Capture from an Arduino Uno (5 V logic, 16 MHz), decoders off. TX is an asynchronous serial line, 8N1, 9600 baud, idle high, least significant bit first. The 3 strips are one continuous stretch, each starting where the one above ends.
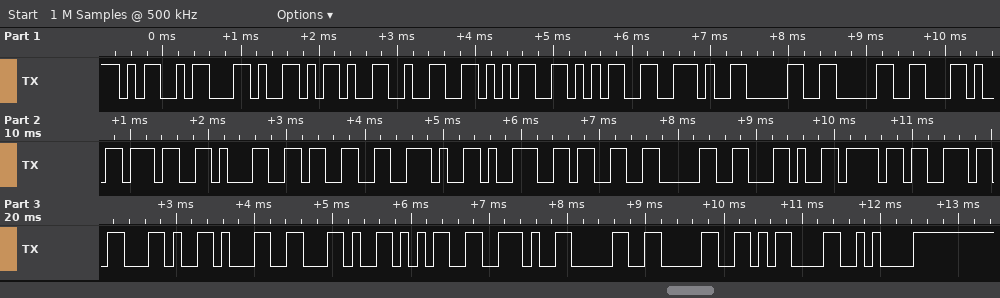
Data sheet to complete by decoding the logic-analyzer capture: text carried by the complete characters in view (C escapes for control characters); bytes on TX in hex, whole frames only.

"M,-255.00,713.930,on,1,5.00\r\n"
4D 2C 2D 32 35 35 2E 30 30 2C 37 31 33 2E 39 33 30 2C 6F 6E 2C 31 2C 35 2E 30 30 0D 0A
